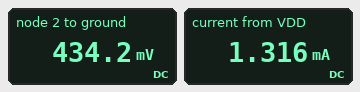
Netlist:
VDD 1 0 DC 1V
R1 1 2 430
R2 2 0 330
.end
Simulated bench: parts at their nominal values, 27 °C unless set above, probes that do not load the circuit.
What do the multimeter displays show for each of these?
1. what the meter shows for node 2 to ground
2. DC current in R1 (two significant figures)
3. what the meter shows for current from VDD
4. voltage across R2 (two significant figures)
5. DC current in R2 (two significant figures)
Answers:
434.2 mV
1.3 mA
1.316 mA
430 mV
1.3 mA
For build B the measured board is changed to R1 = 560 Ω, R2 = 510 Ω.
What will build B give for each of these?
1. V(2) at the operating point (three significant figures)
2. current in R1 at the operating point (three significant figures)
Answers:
477 mV
935 µA
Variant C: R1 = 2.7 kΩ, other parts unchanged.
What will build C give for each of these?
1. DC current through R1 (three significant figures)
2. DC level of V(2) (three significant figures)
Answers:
330 µA
109 mV
